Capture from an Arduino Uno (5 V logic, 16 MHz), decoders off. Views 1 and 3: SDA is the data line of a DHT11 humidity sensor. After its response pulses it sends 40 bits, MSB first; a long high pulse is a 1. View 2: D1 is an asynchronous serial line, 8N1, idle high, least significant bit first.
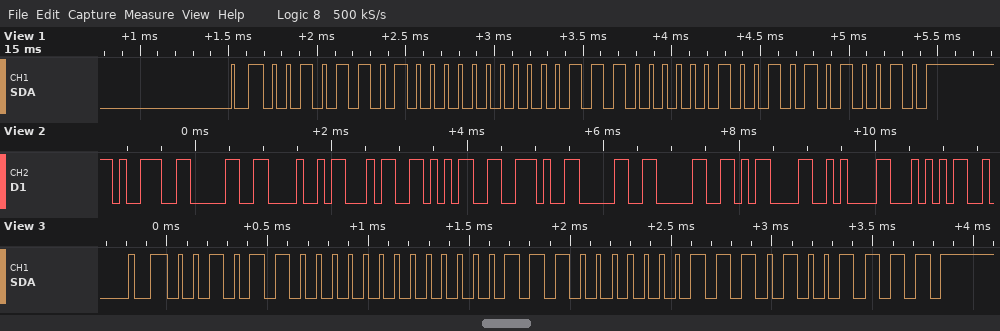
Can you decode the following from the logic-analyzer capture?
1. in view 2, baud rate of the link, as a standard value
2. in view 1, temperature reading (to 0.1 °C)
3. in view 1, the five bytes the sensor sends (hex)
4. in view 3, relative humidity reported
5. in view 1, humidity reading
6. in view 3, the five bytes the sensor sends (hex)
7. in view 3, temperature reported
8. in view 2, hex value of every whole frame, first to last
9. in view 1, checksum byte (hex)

9600 baud
28.9 °C
2D 00 1C 09 52
44 %
45 %
2C 00 1C 07 4F
28.7 °C
39 30 48 34 35 2E 30 30 0D 0A 54
0x52
